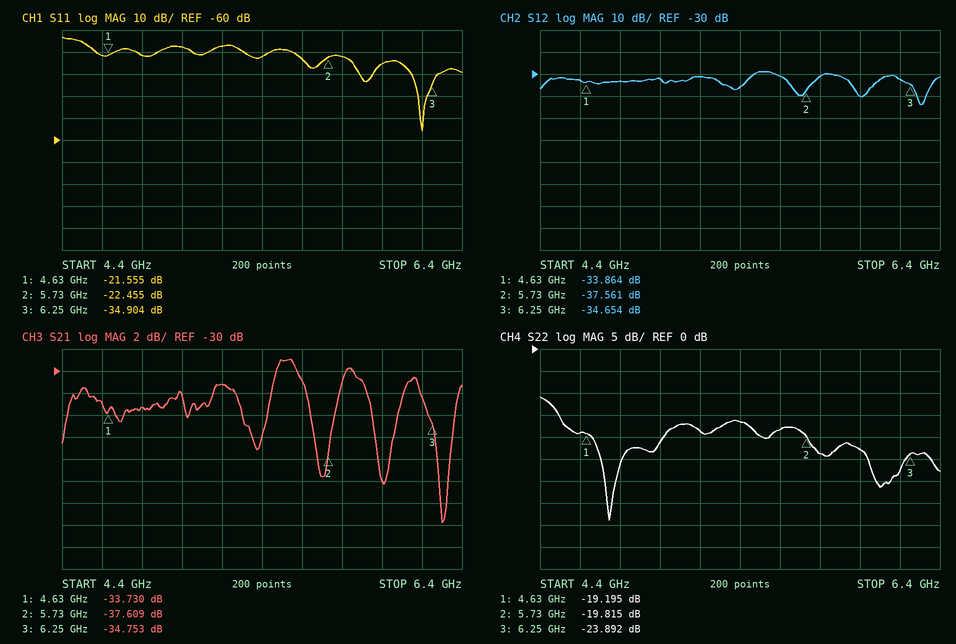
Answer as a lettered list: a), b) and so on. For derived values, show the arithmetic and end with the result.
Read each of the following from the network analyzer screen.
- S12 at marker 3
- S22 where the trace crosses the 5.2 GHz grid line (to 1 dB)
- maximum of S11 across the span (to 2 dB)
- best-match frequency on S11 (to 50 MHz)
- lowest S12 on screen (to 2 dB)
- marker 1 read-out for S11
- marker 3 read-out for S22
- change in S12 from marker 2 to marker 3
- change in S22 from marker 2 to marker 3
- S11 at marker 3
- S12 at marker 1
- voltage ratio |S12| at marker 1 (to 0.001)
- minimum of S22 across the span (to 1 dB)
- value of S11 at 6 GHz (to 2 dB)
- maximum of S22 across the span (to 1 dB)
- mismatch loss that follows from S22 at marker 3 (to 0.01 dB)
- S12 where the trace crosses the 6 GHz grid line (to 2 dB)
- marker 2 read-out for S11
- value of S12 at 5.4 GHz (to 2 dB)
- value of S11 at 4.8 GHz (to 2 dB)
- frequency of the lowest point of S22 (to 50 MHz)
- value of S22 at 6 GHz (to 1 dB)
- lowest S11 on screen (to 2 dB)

a) -34.654 dB
b) -19 dB
c) -14 dB
d) 6.20 GHz
e) -44 dB
f) -21.555 dB
g) -23.892 dB
h) -34.654 − (-37.561) = 2.907 dB
i) -23.892 − (-19.815) = -4.077 dB
j) -34.904 dB
k) -33.864 dB
l) 10^(-33.864/20) ≈ 0.020
m) -39 dB
n) -26 dB
o) -11 dB
p) −10 log10(1 − 10^(-23.892/10)) ≈ 0.02 dB
q) -40 dB
r) -22.455 dB
s) -36 dB
t) -22 dB
u) 4.75 GHz
v) -23 dB
w) -56 dB
